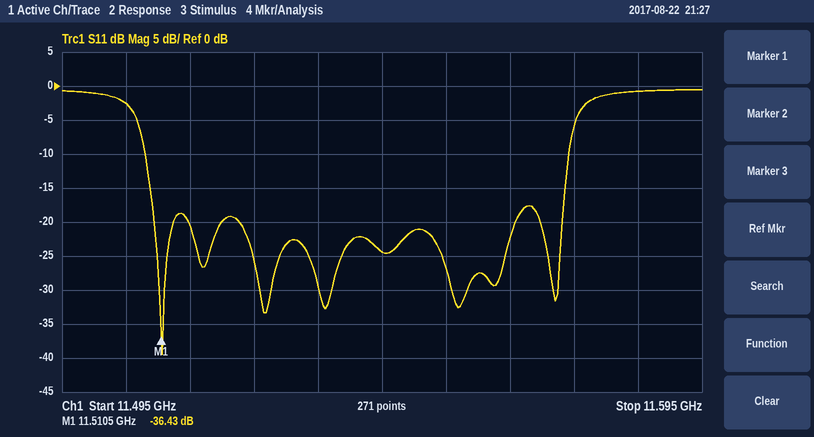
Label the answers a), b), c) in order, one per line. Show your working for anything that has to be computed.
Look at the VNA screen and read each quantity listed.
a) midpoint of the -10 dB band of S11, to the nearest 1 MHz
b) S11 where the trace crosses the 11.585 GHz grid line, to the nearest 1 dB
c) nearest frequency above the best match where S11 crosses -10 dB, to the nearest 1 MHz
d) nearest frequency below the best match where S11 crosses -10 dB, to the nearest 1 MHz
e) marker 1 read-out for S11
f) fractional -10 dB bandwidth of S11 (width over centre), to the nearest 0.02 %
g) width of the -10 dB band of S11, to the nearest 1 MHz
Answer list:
a) 11.541 GHz
b) -1 dB
c) 11.574 GHz
d) 11.508 GHz
e) -36.43 dB
f) 66 MHz / 11.541 GHz ≈ 0.572 %, so 0.58 % to the nearest 0.02 %
g) 11.574 GHz − 11.508 GHz = 66 MHz
